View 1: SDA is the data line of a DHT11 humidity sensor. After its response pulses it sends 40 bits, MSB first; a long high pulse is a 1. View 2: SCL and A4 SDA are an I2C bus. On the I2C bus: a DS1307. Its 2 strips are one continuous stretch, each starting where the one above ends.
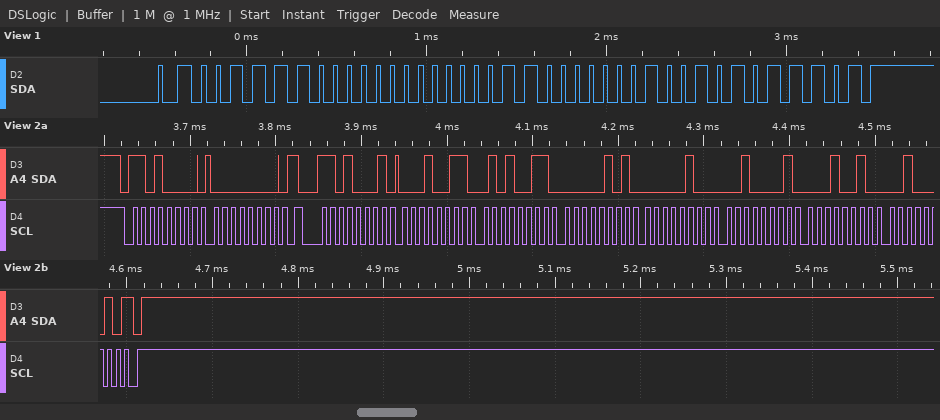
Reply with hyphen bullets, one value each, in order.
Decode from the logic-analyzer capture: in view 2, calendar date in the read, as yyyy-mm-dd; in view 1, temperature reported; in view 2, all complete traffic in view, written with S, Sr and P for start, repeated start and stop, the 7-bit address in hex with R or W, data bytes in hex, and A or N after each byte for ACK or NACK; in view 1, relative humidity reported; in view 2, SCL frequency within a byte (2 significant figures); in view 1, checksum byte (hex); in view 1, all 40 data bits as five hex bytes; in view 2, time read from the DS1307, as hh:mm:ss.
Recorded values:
- 2022-12-21
- 24.9 °C
- S 68W A 00 A Sr 68R A 13 A 53 A 05 A 04 A 21 A 12 A 22 N P
- 60 %
- 100 kHz
- 0x5D
- 3C 00 18 09 5D
- 05:53:13
